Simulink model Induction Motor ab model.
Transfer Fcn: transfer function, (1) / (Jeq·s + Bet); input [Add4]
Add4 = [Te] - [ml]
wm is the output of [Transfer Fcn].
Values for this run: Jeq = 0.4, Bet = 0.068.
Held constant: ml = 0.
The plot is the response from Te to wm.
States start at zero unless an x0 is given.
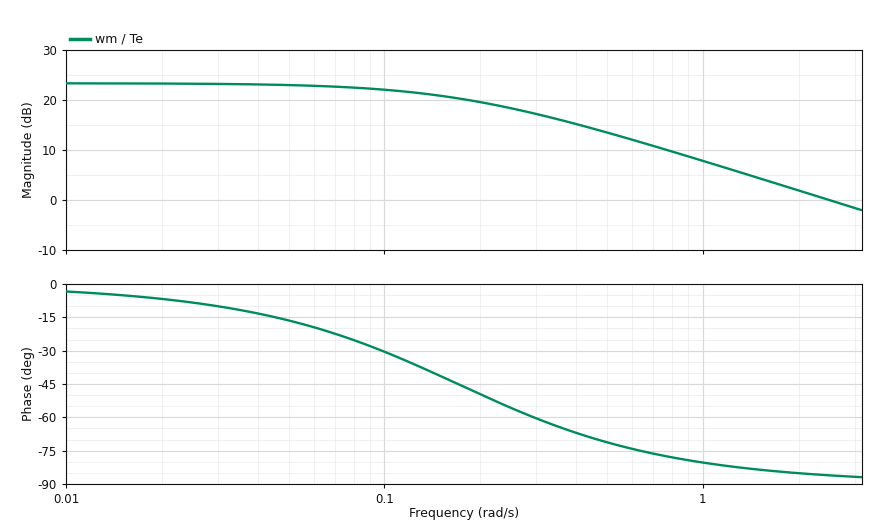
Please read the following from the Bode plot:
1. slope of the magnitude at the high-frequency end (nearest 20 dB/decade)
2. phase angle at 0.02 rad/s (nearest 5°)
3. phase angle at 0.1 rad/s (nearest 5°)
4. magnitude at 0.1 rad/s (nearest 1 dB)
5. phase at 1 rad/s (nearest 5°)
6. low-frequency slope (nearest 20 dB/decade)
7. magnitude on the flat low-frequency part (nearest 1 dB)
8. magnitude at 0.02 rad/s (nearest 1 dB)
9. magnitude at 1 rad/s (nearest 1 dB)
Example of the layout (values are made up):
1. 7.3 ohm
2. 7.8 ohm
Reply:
1. -20 dB/decade
2. -5°
3. -30°
4. 22 dB
5. -80°
6. 0 dB/decade
7. 23 dB
8. 23 dB
9. 8 dB
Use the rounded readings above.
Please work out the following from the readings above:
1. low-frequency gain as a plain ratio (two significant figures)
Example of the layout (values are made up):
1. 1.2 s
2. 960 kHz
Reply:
1. 14
